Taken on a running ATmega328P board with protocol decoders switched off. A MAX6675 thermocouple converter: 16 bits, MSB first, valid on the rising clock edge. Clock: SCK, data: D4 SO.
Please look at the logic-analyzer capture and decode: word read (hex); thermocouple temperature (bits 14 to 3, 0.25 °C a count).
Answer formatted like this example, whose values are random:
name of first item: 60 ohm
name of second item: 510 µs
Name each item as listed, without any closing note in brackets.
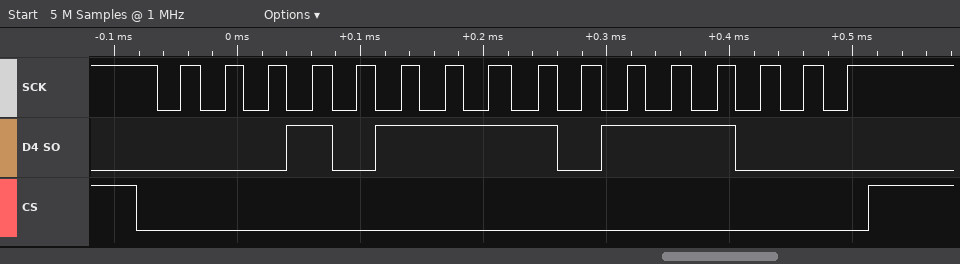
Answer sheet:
word read: 0x17B8
thermocouple temperature: 189.75 °C
